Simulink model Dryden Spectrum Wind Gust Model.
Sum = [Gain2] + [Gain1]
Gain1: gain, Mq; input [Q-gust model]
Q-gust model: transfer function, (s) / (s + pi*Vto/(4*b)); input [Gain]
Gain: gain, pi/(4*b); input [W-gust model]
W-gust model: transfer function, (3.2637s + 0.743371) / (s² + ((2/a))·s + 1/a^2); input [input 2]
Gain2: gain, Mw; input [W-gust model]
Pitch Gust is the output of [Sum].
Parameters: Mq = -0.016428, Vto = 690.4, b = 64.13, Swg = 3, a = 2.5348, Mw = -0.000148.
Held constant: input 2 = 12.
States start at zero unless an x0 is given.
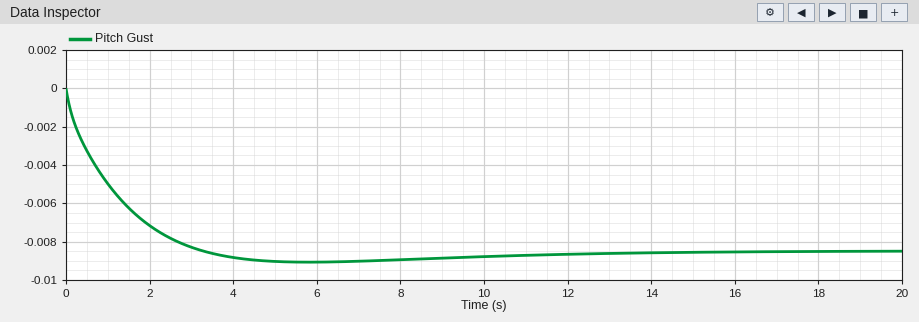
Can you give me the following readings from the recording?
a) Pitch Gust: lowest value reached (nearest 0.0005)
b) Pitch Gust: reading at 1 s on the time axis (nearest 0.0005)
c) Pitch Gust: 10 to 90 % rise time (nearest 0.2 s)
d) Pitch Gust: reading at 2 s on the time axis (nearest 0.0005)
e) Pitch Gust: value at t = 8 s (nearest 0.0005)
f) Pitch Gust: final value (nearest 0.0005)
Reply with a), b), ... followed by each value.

a) -0.0090
b) -0.0050
c) 2.2 s
d) -0.0070
e) -0.0090
f) -0.0085
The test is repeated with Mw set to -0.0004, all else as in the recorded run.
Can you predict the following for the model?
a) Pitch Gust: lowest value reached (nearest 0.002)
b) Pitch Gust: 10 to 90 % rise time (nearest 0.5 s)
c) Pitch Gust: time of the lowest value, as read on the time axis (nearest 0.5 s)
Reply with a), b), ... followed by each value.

a) -0.024
b) 2.5 s
c) 6.0 s
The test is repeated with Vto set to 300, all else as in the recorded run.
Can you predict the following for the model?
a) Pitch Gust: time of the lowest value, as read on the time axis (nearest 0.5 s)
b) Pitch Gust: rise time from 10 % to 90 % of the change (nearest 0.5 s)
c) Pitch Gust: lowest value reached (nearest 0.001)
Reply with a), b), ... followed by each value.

a) 5.5 s
b) 2.0 s
c) -0.009
